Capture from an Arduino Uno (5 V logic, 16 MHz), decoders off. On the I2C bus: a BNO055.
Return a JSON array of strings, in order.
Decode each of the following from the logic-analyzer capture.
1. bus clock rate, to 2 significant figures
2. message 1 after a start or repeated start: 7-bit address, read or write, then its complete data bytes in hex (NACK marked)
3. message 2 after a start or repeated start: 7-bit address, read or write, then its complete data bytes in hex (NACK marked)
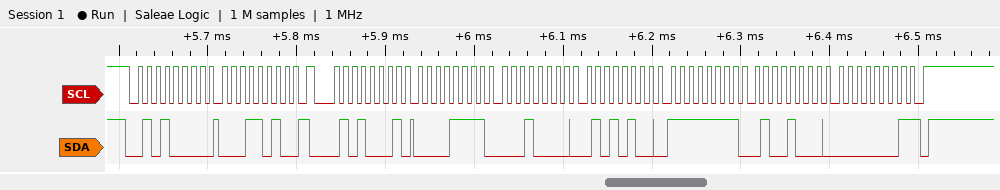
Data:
["100 kHz", "0x28 write: 1A", "0x28 read: 0F 10 54 FF 48 01 NACK"]
